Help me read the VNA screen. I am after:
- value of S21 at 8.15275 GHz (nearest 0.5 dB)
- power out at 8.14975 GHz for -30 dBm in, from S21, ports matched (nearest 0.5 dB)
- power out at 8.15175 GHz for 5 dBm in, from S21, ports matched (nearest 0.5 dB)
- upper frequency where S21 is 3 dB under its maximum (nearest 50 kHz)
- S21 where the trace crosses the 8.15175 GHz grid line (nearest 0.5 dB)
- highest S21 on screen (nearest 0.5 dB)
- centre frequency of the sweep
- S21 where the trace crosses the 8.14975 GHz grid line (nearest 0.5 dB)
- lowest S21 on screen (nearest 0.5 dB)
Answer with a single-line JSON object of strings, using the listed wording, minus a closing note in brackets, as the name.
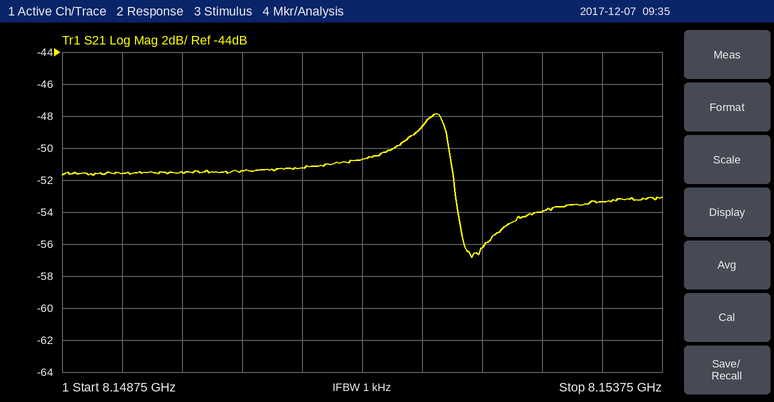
{"value of S21 at 8.15275 GHz": "-54.0 dB", "power out at 8.14975 GHz for -30 dBm in, from S21, ports matched": "-81.5 dBm", "power out at 8.15175 GHz for 5 dBm in, from S21, ports matched": "-43.5 dBm", "upper frequency where S21 is 3 dB under its maximum": "8.15200 GHz", "S21 where the trace crosses the 8.15175 GHz grid line": "-48.5 dB", "highest S21 on screen": "-48.0 dB", "centre frequency of the sweep": "8.15125 GHz", "S21 where the trace crosses the 8.14975 GHz grid line": "-51.5 dB", "lowest S21 on screen": "-57.0 dB"}
